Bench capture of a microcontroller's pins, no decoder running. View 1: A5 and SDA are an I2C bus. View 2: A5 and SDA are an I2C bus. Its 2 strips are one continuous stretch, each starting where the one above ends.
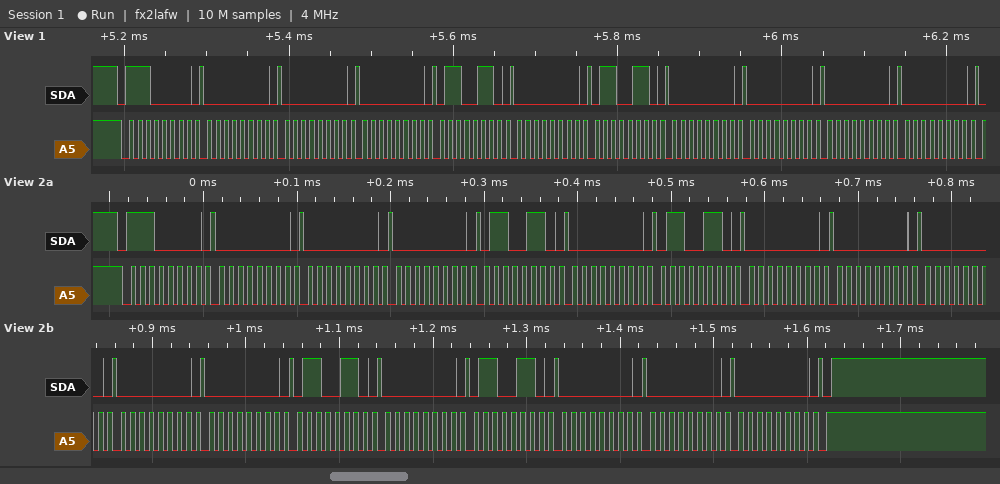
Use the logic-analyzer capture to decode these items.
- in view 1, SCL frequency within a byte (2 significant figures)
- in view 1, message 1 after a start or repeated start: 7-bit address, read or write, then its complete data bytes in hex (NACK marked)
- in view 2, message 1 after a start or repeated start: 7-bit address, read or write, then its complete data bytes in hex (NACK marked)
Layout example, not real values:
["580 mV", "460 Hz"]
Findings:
["100 kHz", "0x70 write: 00 00 00 66 00 66 00 00 00 00", "0x70 write: 00 00 00 66 00 66 00 00 00 00 00 66 00 66 00 00 00"]
